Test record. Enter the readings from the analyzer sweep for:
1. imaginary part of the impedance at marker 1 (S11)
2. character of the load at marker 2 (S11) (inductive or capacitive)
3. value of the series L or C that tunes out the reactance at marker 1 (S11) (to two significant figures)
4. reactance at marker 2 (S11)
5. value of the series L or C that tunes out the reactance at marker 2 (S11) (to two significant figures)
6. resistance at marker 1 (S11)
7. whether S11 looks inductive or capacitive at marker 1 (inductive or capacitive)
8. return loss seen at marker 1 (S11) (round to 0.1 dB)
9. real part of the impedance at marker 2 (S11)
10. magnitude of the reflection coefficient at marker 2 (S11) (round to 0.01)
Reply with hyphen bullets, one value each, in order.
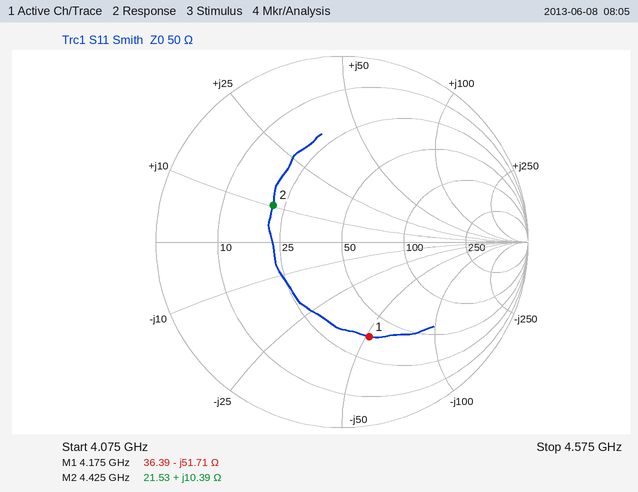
- -51.71 Ω
- inductive
- 2.0 nH
- +10.39 Ω
- 3.5 pF
- 36.39 Ω
- capacitive
- 5.5 dB
- 21.53 Ω
- 0.42
